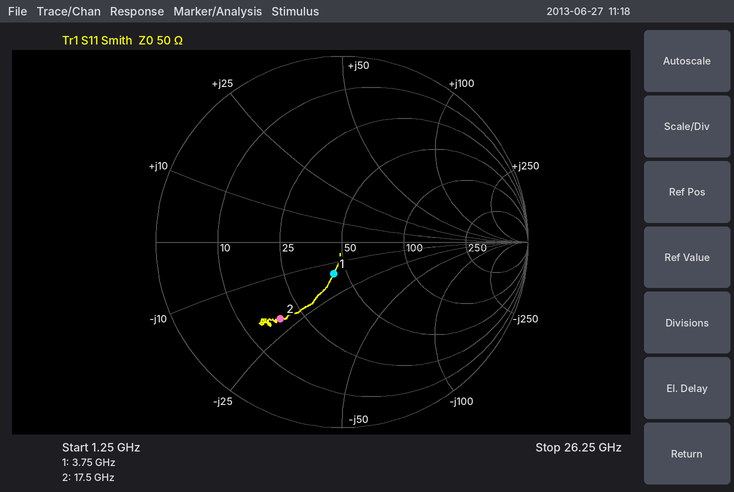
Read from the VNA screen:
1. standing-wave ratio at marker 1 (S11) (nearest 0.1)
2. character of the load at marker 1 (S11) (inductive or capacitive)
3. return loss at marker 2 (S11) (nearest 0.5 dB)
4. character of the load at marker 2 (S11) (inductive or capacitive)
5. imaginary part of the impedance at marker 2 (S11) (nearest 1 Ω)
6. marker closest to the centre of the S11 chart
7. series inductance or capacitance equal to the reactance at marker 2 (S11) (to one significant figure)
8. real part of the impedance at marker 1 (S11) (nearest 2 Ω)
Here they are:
1.4
capacitive
5.5 dB
capacitive
-21 Ω
marker 1
400 fF
44 Ω
